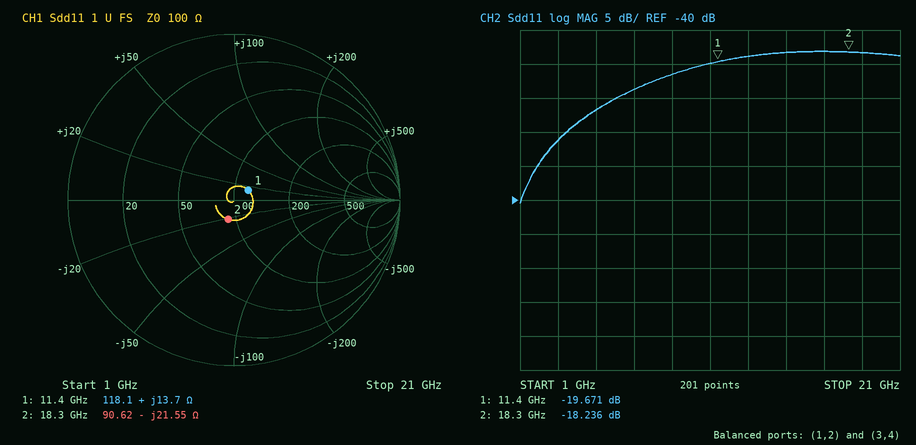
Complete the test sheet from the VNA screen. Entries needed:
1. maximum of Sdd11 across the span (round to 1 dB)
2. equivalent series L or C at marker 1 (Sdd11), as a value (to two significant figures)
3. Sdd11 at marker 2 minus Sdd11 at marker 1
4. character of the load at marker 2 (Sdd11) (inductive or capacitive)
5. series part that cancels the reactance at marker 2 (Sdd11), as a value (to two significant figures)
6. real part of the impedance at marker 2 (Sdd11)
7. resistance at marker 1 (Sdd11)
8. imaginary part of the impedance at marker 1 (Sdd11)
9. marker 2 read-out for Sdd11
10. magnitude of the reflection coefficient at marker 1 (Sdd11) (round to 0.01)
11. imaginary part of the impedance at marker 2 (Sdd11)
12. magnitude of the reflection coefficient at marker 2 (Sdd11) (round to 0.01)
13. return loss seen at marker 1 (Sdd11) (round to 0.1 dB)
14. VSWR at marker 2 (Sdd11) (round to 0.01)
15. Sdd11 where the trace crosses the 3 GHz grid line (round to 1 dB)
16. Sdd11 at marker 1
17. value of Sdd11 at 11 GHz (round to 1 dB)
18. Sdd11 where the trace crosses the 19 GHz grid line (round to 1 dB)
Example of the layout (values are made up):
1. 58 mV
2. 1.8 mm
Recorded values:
1. -18 dB
2. 190 pH
3. 1.435 dB
4. capacitive
5. 190 pH
6. 90.62 Ω
7. 118.1 Ω
8. +13.7 Ω
9. -18.236 dB
10. 0.10
11. -21.55 Ω
12. 0.12
13. 19.7 dB
14. 1.28
15. -31 dB
16. -19.671 dB
17. -20 dB
18. -18 dB
